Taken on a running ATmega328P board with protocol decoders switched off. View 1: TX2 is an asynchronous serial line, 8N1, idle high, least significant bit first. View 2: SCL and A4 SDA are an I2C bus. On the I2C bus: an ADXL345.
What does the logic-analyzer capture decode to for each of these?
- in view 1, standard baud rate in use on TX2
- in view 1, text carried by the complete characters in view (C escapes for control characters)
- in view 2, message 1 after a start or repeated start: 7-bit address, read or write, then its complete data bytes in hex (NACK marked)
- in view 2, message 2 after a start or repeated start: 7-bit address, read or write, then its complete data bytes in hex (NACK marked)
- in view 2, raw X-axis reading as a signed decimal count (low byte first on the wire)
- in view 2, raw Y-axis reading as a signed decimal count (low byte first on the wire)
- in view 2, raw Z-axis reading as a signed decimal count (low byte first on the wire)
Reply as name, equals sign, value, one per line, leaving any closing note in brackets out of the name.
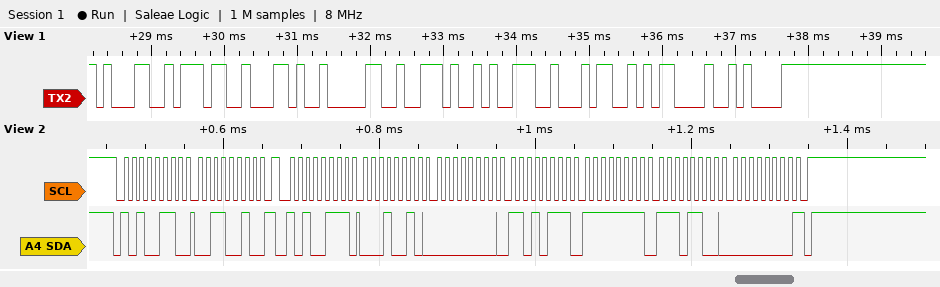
in view 1, standard baud rate in use on TX2 = 9600 baud
in view 1, text carried by the complete characters in view = "17,0.94\r\n"
in view 2, message 1 after a start or repeated start: 7-bit address, read or write, then its complete data bytes in hex = 0x53 write: 32
in view 2, message 2 after a start or repeated start: 7-bit address, read or write, then its complete data bytes in hex = 0x53 read: 12 00 D7 FF EC 00 NACK
in view 2, raw X-axis reading as a signed decimal count = 18
in view 2, raw Y-axis reading as a signed decimal count = -41
in view 2, raw Z-axis reading as a signed decimal count = 236
